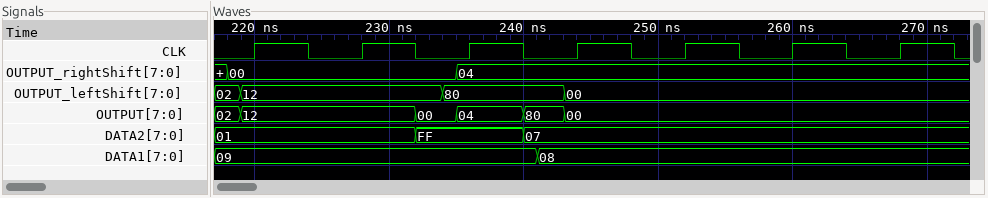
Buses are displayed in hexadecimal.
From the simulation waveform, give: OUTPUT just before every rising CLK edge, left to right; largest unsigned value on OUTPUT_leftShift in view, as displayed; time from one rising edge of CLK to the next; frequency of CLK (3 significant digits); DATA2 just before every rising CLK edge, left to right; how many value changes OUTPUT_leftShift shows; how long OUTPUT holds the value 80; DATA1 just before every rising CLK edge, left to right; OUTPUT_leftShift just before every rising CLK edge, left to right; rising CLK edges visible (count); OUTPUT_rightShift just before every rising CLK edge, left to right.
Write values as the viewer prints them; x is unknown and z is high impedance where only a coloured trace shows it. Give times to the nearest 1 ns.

12, 12, 04, 00, 00, 00, 00
80
8 ns
125 MHz
01, 01, FF, 07, 07, 07, 07
3
3 ns
09, 09, 09, 08, 08, 08, 08
12, 12, 80, 00, 00, 00, 00
7
00, 00, 04, 04, 04, 04, 04
